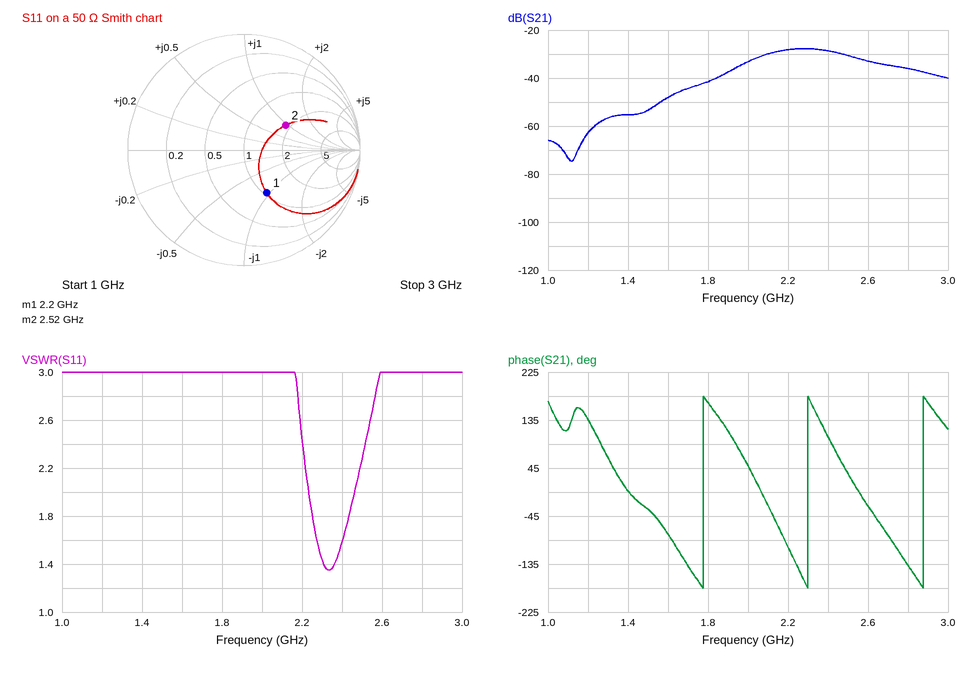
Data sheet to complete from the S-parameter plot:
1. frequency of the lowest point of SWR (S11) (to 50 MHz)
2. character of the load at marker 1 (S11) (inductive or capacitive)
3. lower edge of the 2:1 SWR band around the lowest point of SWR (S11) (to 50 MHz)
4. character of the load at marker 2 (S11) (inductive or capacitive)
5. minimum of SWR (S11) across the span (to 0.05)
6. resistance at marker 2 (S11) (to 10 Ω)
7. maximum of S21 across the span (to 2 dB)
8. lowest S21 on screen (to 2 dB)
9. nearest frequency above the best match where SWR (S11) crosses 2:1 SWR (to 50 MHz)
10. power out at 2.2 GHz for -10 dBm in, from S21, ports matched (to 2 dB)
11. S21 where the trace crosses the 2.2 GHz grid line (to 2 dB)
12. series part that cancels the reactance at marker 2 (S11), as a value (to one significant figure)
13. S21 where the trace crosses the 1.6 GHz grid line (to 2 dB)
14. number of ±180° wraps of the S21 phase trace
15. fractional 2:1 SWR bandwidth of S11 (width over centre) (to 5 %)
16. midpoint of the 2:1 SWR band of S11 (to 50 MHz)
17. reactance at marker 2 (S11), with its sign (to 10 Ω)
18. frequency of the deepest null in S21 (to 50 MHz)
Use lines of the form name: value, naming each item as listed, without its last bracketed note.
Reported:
frequency of the lowest point of SWR (S11): 2.35 GHz
character of the load at marker 1 (S11): capacitive
lower edge of the 2:1 SWR band around the lowest point of SWR (S11): 2.25 GHz
character of the load at marker 2 (S11): inductive
minimum of SWR (S11) across the span: 1.35
resistance at marker 2 (S11): 90 Ω
maximum of S21 across the span: -28 dB
lowest S21 on screen: -74 dB
nearest frequency above the best match where SWR (S11) crosses 2:1 SWR: 2.45 GHz
power out at 2.2 GHz for -10 dBm in, from S21, ports matched: -38 dBm
S21 where the trace crosses the 2.2 GHz grid line: -28 dB
series part that cancels the reactance at marker 2 (S11), as a value: 1 pF
S21 where the trace crosses the 1.6 GHz grid line: -48 dB
number of ±180° wraps of the S21 phase trace: 3
fractional 2:1 SWR bandwidth of S11 (width over centre): 10 %
midpoint of the 2:1 SWR band of S11: 2.35 GHz
reactance at marker 2 (S11), with its sign: +50 Ω
frequency of the deepest null in S21: 1.10 GHz
